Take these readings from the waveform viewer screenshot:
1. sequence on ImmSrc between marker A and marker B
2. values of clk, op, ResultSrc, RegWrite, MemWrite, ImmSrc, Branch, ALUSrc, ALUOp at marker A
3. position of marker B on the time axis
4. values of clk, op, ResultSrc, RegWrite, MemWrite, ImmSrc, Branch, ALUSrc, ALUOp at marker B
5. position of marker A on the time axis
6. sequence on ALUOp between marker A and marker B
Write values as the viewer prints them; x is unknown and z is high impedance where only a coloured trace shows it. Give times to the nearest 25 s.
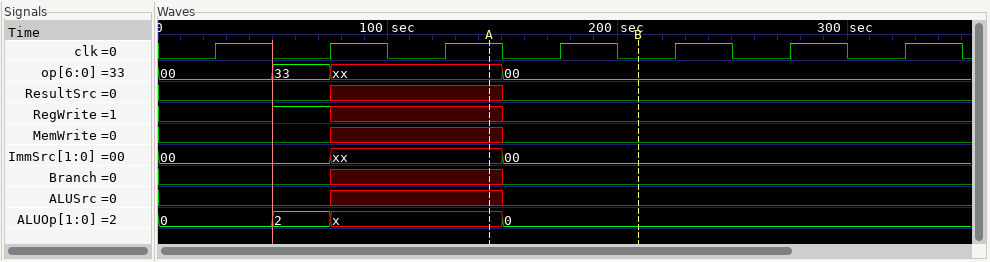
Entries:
xx, 00
clk=1, op=xx, ResultSrc=x, RegWrite=x, MemWrite=x, ImmSrc=xx, Branch=x, ALUSrc=x, ALUOp=x
200 s
clk=0, op=00, ResultSrc=0, RegWrite=0, MemWrite=0, ImmSrc=00, Branch=0, ALUSrc=0, ALUOp=0
150 s
x, 0
